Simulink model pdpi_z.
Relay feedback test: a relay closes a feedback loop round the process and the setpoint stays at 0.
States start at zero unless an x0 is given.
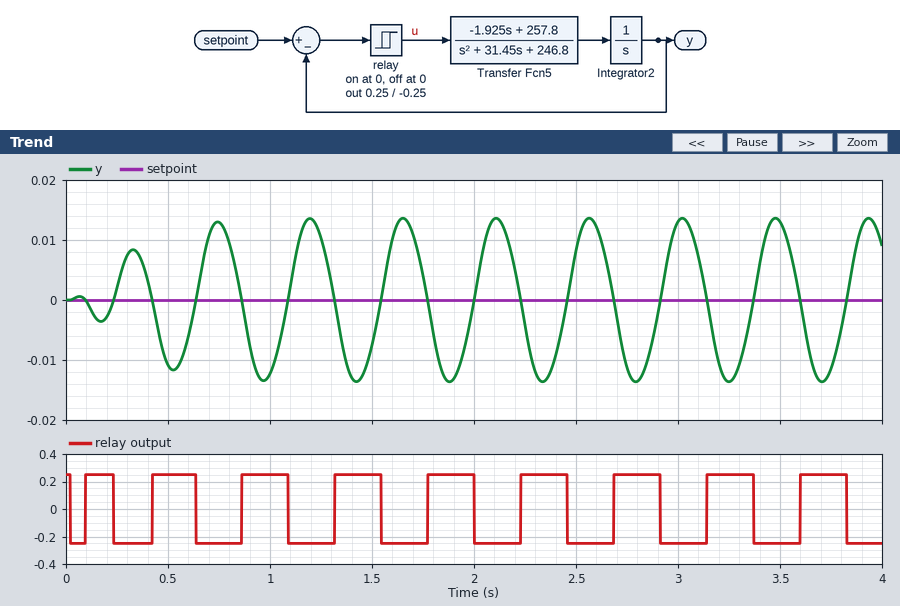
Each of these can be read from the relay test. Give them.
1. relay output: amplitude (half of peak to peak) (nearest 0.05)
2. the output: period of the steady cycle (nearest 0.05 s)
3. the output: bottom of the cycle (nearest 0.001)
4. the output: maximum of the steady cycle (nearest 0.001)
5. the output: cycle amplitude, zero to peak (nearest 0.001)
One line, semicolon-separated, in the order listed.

0.25; 0.45 s; -0.014; 0.014; 0.014
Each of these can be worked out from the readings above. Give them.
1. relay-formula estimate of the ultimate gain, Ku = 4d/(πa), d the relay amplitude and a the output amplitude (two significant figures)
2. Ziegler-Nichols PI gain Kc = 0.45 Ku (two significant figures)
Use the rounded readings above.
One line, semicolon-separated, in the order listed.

23; 10
